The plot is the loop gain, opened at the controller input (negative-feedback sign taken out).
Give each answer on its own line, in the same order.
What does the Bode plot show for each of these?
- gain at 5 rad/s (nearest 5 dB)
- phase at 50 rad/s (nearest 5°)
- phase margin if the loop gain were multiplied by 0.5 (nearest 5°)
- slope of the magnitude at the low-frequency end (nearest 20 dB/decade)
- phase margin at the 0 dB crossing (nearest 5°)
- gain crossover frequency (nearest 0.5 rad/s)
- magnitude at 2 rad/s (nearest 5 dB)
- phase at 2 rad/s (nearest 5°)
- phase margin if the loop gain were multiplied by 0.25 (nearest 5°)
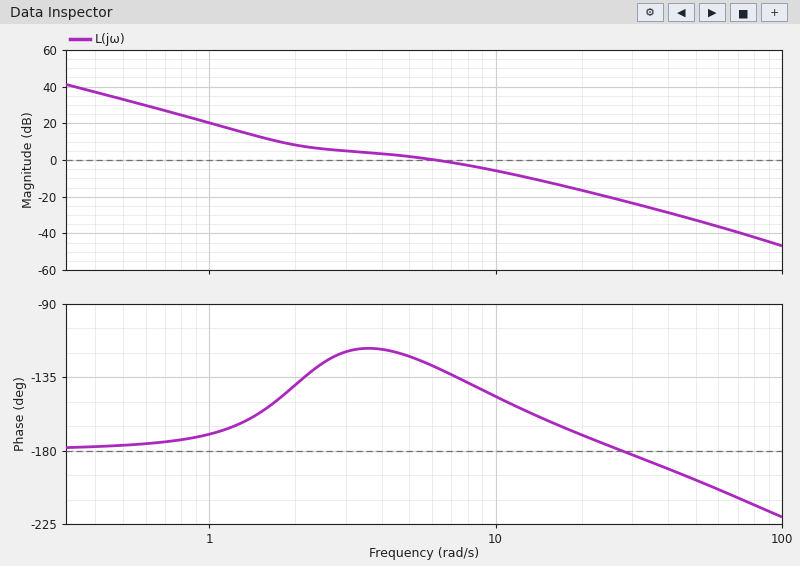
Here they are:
0 dB
-200°
55°
-40 dB/decade
50°
6.0 rad/s
10 dB
-140°
25°
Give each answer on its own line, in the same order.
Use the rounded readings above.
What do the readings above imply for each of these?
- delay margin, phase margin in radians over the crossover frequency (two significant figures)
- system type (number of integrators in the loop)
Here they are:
0.15 s
2
